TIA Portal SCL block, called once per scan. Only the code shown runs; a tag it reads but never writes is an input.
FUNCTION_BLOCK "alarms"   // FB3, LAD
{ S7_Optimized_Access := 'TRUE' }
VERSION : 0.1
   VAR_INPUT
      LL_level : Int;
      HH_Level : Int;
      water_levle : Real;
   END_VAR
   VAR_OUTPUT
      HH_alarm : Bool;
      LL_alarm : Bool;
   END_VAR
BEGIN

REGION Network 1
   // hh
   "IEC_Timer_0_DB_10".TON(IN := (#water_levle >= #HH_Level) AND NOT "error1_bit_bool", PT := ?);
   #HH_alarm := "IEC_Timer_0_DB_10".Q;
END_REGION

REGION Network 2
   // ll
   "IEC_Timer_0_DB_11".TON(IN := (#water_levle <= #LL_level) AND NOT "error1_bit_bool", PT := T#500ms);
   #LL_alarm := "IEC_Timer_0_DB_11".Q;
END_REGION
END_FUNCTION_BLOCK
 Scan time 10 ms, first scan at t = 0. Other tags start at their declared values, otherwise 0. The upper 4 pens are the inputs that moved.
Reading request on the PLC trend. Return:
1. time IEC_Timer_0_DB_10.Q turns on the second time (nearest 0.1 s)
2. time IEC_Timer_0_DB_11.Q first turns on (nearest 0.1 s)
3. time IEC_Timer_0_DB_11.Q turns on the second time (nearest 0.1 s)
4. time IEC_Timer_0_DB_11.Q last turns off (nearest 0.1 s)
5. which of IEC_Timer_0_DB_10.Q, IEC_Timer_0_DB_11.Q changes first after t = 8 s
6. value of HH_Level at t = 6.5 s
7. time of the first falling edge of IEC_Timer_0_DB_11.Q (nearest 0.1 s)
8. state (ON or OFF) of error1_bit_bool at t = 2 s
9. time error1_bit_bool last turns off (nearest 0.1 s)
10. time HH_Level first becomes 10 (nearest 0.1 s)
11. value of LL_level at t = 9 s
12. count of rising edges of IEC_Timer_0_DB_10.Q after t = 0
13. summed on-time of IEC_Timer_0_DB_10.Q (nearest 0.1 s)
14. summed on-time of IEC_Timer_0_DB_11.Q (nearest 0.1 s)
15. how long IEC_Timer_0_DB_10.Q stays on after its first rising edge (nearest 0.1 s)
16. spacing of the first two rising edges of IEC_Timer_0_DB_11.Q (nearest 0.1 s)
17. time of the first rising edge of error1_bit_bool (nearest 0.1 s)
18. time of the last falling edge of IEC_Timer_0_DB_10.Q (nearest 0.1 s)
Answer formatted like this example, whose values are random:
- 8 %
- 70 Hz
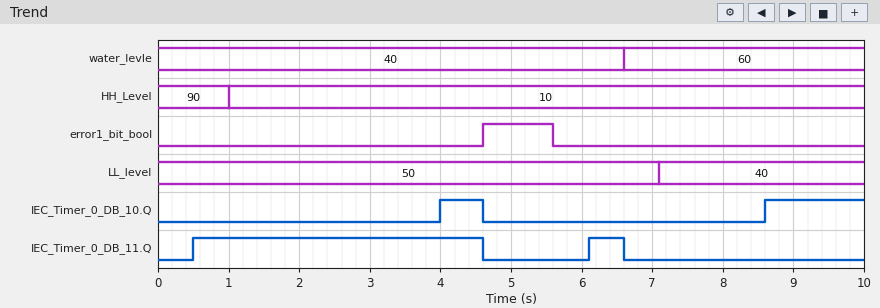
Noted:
- 8.6 s
- 0.5 s
- 6.1 s
- 6.6 s
- IEC_Timer_0_DB_10.Q
- 10
- 4.6 s
- OFF
- 5.6 s
- 1.0 s
- 40
- 2
- 2.0 s
- 4.6 s
- 0.6 s
- 5.6 s
- 4.6 s
- 4.6 s
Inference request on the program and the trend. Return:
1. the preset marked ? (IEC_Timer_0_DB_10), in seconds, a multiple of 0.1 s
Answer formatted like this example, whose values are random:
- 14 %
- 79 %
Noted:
- 3.0 s
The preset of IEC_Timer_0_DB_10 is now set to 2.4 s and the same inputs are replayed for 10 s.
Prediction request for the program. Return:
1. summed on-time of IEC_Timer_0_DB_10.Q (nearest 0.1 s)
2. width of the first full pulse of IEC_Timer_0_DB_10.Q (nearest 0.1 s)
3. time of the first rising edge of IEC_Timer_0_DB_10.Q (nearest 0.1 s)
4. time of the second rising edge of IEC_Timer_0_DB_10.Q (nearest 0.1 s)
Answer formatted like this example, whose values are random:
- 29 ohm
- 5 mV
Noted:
- 3.2 s
- 1.2 s
- 3.4 s
- 8.0 s
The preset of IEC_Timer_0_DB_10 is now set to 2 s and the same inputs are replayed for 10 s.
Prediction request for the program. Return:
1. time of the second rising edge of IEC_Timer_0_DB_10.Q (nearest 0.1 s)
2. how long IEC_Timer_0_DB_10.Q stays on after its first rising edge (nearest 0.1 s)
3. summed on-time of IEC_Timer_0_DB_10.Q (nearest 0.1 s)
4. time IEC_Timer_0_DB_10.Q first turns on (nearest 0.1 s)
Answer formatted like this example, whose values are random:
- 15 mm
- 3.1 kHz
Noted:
- 7.6 s
- 1.6 s
- 4.0 s
- 3.0 s
